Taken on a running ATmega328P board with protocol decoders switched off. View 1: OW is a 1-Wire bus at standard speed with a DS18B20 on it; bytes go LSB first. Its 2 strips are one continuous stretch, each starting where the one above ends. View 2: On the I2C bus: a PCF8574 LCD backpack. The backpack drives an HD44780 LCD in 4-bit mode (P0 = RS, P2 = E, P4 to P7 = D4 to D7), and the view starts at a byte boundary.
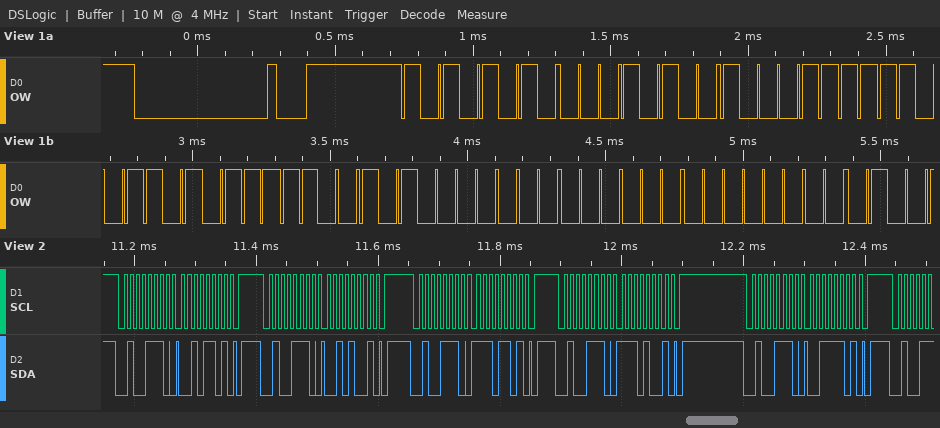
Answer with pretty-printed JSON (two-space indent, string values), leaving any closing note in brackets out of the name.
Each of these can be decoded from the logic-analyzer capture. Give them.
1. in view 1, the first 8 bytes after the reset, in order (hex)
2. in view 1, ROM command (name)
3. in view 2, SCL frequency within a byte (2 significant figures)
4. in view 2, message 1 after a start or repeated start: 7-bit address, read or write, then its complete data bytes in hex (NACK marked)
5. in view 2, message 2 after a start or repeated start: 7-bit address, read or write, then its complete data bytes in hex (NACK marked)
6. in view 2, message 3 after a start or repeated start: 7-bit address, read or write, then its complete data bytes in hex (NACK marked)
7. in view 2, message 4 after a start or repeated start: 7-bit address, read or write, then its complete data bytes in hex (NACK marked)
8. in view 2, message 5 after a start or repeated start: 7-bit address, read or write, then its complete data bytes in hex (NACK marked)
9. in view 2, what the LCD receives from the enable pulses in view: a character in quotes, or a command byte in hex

{
  "in view 1, the first 8 bytes after the reset, in order": "55 28 F1 B3 3E 05 00 00",
  "in view 1, ROM command": "Match ROM",
  "in view 2, SCL frequency within a byte": "100 kHz",
  "in view 2, message 1 after a start or repeated start: 7-bit address, read or write, then its complete data bytes in hex": "0x27 write: 2D",
  "in view 2, message 2 after a start or repeated start: 7-bit address, read or write, then its complete data bytes in hex": "0x27 write: 29",
  "in view 2, message 3 after a start or repeated start: 7-bit address, read or write, then its complete data bytes in hex": "0x27 write: ED",
  "in view 2, message 4 after a start or repeated start: 7-bit address, read or write, then its complete data bytes in hex": "0x27 write: E9",
  "in view 2, message 5 after a start or repeated start: 7-bit address, read or write, then its complete data bytes in hex": "0x27 write: 3D",
  "in view 2, what the LCD receives from the enable pulses in view: a character in quotes, or a command byte in hex": "'.'"
}
